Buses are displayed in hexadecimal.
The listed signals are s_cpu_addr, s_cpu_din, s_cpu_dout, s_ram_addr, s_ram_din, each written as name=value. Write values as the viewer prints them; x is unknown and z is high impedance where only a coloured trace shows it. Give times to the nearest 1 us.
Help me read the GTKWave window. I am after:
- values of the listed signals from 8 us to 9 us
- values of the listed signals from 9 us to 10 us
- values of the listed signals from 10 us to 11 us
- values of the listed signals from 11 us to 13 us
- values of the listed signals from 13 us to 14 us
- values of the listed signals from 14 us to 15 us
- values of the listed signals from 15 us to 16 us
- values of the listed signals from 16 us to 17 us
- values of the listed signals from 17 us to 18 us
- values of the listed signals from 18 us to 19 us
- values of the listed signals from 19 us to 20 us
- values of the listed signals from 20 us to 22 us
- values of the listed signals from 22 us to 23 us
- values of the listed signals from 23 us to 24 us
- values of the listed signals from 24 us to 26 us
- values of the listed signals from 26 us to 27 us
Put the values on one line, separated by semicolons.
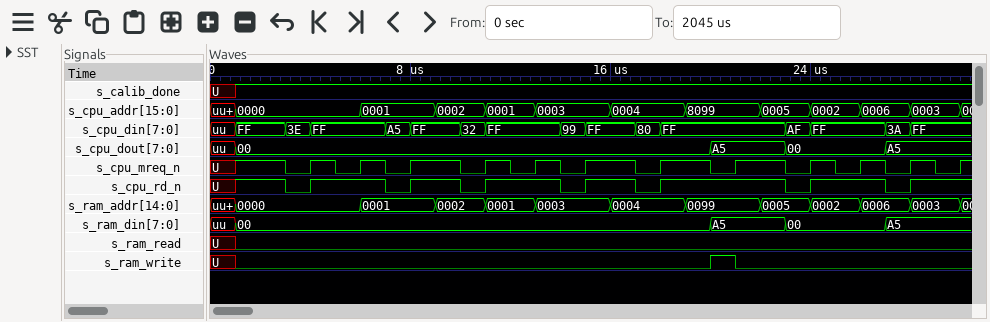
s_cpu_addr=0001, s_cpu_din=FF, s_cpu_dout=00, s_ram_addr=0001, s_ram_din=00; s_cpu_addr=0002, s_cpu_din=FF, s_cpu_dout=00, s_ram_addr=0002, s_ram_din=00; s_cpu_addr=0002, s_cpu_din=32, s_cpu_dout=00, s_ram_addr=0002, s_ram_din=00; s_cpu_addr=0001, s_cpu_din=FF, s_cpu_dout=00, s_ram_addr=0001, s_ram_din=00; s_cpu_addr=0003, s_cpu_din=FF, s_cpu_dout=00, s_ram_addr=0003, s_ram_din=00; s_cpu_addr=0003, s_cpu_din=99, s_cpu_dout=00, s_ram_addr=0003, s_ram_din=00; s_cpu_addr=0003, s_cpu_din=FF, s_cpu_dout=00, s_ram_addr=0003, s_ram_din=00; s_cpu_addr=0004, s_cpu_din=FF, s_cpu_dout=00, s_ram_addr=0004, s_ram_din=00; s_cpu_addr=0004, s_cpu_din=80, s_cpu_dout=00, s_ram_addr=0004, s_ram_din=00; s_cpu_addr=0004, s_cpu_din=FF, s_cpu_dout=00, s_ram_addr=0004, s_ram_din=00; s_cpu_addr=8099, s_cpu_din=FF, s_cpu_dout=00, s_ram_addr=0099, s_ram_din=00; s_cpu_addr=8099, s_cpu_din=FF, s_cpu_dout=A5, s_ram_addr=0099, s_ram_din=A5; s_cpu_addr=0005, s_cpu_din=FF, s_cpu_dout=A5, s_ram_addr=0005, s_ram_din=A5; s_cpu_addr=0005, s_cpu_din=AF, s_cpu_dout=00, s_ram_addr=0005, s_ram_din=00; s_cpu_addr=0002, s_cpu_din=FF, s_cpu_dout=00, s_ram_addr=0002, s_ram_din=00; s_cpu_addr=0006, s_cpu_din=FF, s_cpu_dout=00, s_ram_addr=0006, s_ram_din=00
